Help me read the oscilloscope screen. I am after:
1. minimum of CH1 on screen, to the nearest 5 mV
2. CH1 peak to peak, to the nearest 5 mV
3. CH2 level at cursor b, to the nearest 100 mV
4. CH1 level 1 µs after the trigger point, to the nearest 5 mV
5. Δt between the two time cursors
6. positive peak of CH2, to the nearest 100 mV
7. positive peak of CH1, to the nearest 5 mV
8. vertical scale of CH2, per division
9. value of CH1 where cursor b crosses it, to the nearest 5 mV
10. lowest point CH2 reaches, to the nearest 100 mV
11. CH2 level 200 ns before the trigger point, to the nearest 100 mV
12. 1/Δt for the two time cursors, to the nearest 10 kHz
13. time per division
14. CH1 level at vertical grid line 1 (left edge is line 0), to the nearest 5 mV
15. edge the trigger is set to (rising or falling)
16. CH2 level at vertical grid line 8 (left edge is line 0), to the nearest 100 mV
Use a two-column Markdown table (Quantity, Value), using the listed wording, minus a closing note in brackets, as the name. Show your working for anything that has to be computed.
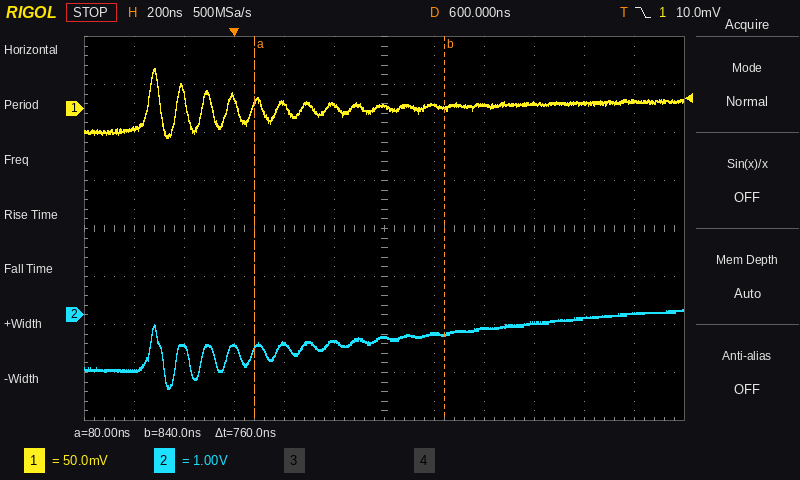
| Quantity | Value |
|---|---|
| minimum of CH1 on screen, to the nearest 5 mV | -30 mV |
| CH1 peak to peak, to the nearest 5 mV | 40 mV − (-30 mV) = 70 mV |
| CH2 level at cursor b, to the nearest 100 mV | -400 mV |
| CH1 level 1 µs after the trigger point, to the nearest 5 mV | 5 mV |
| Δt between the two time cursors | 760 ns |
| positive peak of CH2, to the nearest 100 mV | 100 mV |
| positive peak of CH1, to the nearest 5 mV | 40 mV |
| vertical scale of CH2, per division | 1 V |
| value of CH1 where cursor b crosses it, to the nearest 5 mV | 0 mV |
| lowest point CH2 reaches, to the nearest 100 mV | -1.5 V |
| CH2 level 200 ns before the trigger point, to the nearest 100 mV | -700 mV |
| 1/Δt for the two time cursors, to the nearest 10 kHz | 1 / 760 ns ≈ 1.32 MHz |
| time per division | 200 ns |
| CH1 level at vertical grid line 1 (left edge is line 0), to the nearest 5 mV | -20 mV |
| edge the trigger is set to | falling |
| CH2 level at vertical grid line 8 (left edge is line 0), to the nearest 100 mV | -300 mV |
